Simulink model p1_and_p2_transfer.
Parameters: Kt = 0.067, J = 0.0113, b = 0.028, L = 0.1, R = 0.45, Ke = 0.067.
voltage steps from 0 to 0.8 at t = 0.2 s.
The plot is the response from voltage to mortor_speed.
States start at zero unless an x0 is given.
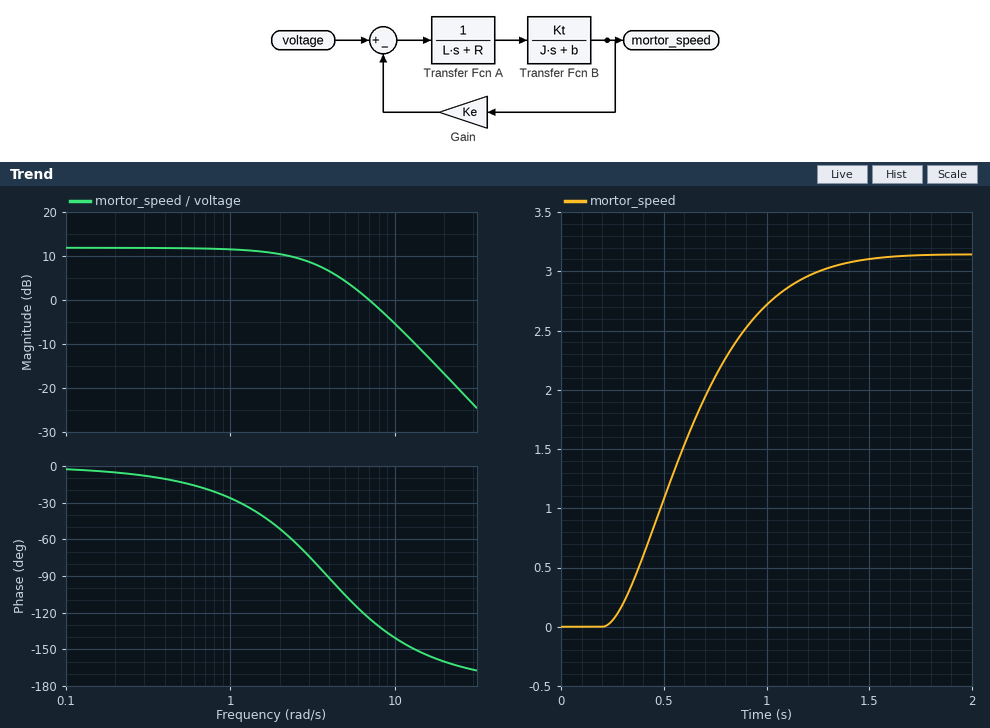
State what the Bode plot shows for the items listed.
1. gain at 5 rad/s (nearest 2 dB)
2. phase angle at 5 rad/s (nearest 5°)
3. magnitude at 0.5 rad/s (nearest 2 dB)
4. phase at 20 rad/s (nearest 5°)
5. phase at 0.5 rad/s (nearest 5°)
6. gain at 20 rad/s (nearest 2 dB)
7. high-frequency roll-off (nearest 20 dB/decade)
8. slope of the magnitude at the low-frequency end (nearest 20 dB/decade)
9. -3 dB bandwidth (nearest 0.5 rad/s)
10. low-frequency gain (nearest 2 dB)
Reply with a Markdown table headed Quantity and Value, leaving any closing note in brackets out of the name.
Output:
| Quantity | Value |
|---|---|
| gain at 5 rad/s | 4 dB |
| phase angle at 5 rad/s | -105° |
| magnitude at 0.5 rad/s | 12 dB |
| phase at 20 rad/s | -160° |
| phase at 0.5 rad/s | -15° |
| gain at 20 rad/s | -16 dB |
| high-frequency roll-off | -40 dB/decade |
| slope of the magnitude at the low-frequency end | 0 dB/decade |
| -3 dB bandwidth | 3.0 rad/s |
| low-frequency gain | 12 dB |
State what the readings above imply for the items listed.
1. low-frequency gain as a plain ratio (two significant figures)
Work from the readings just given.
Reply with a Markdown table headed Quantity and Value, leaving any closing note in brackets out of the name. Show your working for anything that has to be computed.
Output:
| Quantity | Value |
|---|---|
| low-frequency gain as a plain ratio | 10^(12 / 20) = 4.0 |
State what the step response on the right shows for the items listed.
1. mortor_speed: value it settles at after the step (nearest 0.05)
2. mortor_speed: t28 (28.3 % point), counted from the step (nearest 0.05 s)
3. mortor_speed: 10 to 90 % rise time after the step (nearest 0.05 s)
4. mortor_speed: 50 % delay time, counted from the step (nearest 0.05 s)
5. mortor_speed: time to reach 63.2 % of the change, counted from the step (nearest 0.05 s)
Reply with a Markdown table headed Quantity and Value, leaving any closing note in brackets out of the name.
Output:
| Quantity | Value |
|---|---|
| mortor_speed: value it settles at after the step | 3.15 |
| mortor_speed: t28 (28.3 % point), counted from the step | 0.25 s |
| mortor_speed: 10 to 90 % rise time after the step | 0.75 s |
| mortor_speed: 50 % delay time, counted from the step | 0.40 s |
| mortor_speed: time to reach 63.2 % of the change, counted from the step | 0.50 s |
